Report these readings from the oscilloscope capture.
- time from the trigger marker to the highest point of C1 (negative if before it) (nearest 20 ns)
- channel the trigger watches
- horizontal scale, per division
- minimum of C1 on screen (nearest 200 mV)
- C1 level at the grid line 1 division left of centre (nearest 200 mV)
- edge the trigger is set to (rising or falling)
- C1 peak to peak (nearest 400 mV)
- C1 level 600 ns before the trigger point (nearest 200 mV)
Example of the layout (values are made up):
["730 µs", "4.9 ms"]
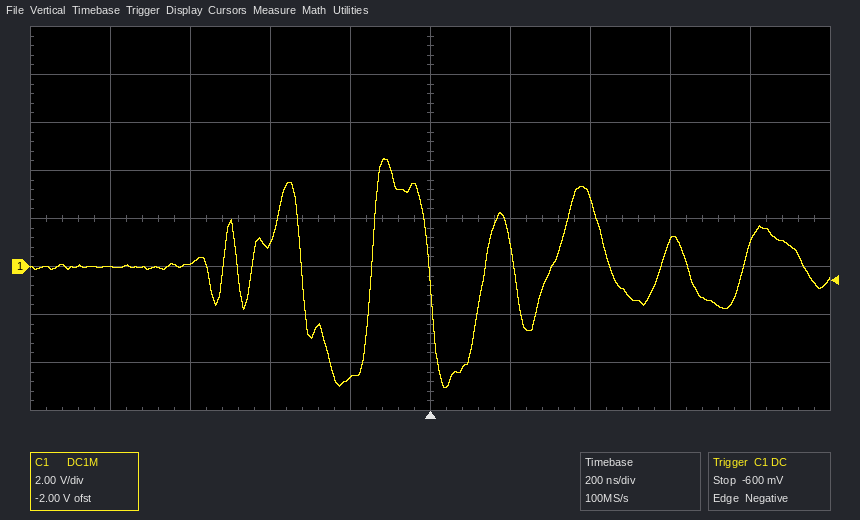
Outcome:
["-120 ns", "C1", "200 ns", "-5.0 V", "-4.6 V", "falling", "9.6 V", "200 mV"]
